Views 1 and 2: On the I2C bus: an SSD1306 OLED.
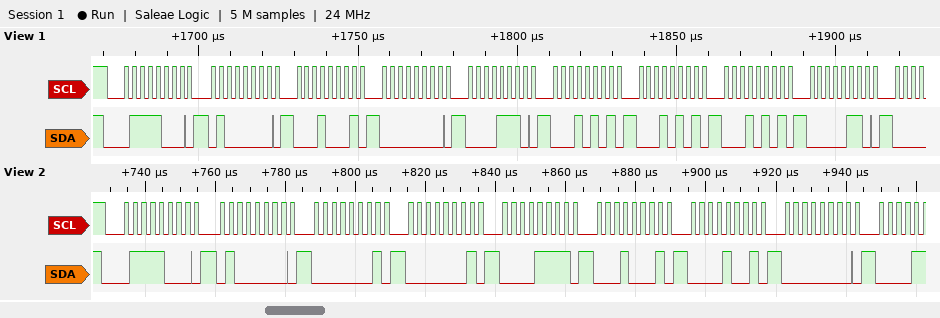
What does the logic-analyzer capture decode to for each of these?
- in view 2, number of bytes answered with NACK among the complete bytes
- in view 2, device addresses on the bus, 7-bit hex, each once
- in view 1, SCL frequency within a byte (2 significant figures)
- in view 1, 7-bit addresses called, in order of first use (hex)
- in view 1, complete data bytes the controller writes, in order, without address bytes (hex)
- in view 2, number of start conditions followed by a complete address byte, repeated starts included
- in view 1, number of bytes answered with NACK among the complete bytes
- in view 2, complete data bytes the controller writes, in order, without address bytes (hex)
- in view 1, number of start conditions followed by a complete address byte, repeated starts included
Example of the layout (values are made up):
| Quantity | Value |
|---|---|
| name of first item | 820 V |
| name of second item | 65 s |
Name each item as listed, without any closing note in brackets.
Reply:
| Quantity | Value |
|---|---|
| in view 2, number of bytes answered with NACK among the complete bytes | 0 |
| in view 2, device addresses on the bus, 7-bit hex, each once | 0x3C |
| in view 1, SCL frequency within a byte | 400 kHz |
| in view 1, 7-bit addresses called, in order of first use | 0x3C |
| in view 1, complete data bytes the controller writes, in order, without address bytes | 40 11 00 0E 15 15 15 06 |
| in view 2, number of start conditions followed by a complete address byte, repeated starts included | 1 |
| in view 1, number of bytes answered with NACK among the complete bytes | 0 |
| in view 2, complete data bytes the controller writes, in order, without address bytes | 40 01 01 0F 11 09 00 |
| in view 1, number of start conditions followed by a complete address byte, repeated starts included | 1 |
